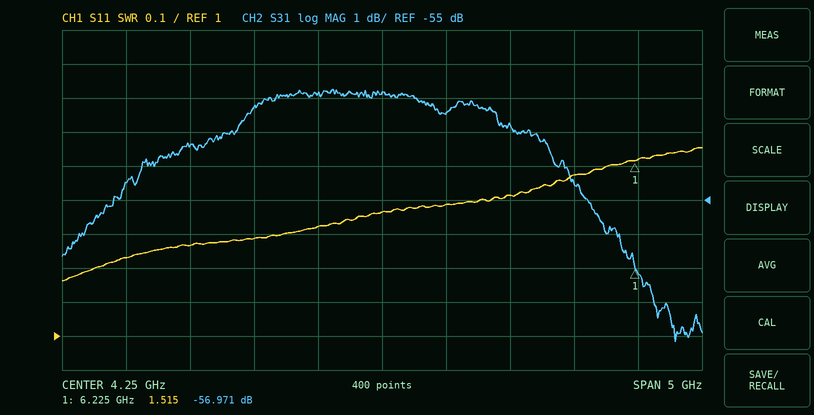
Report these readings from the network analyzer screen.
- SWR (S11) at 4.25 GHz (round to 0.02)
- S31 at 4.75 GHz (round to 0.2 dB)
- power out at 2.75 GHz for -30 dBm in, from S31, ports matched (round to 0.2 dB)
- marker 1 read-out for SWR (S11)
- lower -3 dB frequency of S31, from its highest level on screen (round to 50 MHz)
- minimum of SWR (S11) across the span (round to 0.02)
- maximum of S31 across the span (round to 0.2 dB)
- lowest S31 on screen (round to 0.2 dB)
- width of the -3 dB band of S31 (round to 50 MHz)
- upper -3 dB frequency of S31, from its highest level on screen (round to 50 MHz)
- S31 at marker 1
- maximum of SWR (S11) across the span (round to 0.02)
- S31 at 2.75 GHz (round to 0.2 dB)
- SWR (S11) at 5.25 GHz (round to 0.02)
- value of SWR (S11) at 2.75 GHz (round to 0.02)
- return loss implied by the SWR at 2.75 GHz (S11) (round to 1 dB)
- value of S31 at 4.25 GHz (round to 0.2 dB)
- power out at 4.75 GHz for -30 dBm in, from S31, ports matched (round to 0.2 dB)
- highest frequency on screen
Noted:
1.36
-52.4 dB
-83.4 dBm
1.515
2.20 GHz
1.16
-51.8 dB
-59.2 dB
3.60 GHz
5.80 GHz
-56.971 dB
1.56
-53.4 dB
1.42
1.26
19 dB
-51.8 dB
-82.4 dBm
6.75 GHz
